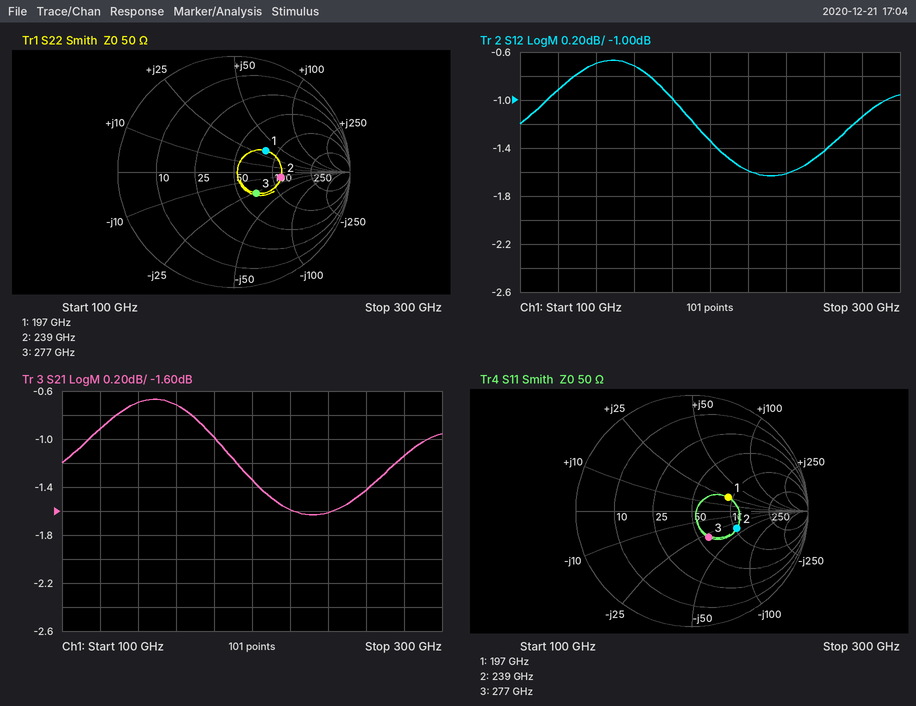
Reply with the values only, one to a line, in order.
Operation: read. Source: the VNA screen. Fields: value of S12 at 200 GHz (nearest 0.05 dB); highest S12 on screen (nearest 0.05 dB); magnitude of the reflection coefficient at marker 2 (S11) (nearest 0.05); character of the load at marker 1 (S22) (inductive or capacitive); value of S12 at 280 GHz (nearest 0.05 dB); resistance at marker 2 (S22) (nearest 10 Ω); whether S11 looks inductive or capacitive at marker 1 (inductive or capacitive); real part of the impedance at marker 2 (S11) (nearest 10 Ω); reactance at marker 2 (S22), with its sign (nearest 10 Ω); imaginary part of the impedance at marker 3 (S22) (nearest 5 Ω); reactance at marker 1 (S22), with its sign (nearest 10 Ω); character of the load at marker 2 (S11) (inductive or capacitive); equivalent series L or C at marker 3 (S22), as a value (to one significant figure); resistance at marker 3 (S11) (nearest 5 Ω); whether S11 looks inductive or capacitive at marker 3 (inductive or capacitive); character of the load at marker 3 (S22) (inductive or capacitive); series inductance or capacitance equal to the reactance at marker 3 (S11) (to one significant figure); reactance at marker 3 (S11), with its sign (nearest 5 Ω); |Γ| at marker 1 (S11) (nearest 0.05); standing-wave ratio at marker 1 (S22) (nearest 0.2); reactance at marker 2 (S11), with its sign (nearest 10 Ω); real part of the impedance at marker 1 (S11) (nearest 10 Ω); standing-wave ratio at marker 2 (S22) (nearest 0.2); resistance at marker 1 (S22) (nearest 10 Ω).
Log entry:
-1.35 dB
-0.65 dB
0.40
inductive
-1.15 dB
120 Ω
inductive
100 Ω
-10 Ω
-25 Ω
+30 Ω
capacitive
20 fF
60 Ω
capacitive
capacitive
20 fF
-30 Ω
0.35
2.0
-40 Ω
90 Ω
2.4
80 Ω
